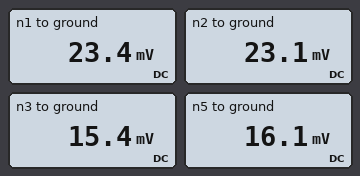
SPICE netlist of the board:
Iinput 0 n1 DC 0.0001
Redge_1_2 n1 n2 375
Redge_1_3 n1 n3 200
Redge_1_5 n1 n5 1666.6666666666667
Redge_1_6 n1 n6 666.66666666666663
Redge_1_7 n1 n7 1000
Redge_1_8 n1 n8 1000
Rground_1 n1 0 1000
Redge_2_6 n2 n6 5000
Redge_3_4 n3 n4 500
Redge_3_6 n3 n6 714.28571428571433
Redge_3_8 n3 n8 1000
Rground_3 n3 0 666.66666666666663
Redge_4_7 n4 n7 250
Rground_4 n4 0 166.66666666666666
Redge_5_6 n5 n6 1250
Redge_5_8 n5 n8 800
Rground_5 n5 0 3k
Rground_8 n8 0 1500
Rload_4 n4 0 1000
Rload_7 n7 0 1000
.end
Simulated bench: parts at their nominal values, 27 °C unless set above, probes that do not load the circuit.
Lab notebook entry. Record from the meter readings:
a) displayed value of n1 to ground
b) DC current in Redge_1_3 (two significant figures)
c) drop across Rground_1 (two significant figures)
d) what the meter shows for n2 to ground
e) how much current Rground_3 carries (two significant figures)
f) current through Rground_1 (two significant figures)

23.4 mV
40 µA
23 mV
23.1 mV
23 µA
23 µA
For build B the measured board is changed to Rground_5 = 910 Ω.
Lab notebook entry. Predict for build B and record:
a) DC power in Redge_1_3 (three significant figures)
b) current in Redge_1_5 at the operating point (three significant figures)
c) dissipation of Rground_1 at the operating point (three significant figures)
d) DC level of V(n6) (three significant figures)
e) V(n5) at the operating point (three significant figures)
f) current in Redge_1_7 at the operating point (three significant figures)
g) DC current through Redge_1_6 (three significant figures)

301 nW
6.31 µA
482 nW
17.0 mV
11.4 mV
15.5 µA
7.44 µA
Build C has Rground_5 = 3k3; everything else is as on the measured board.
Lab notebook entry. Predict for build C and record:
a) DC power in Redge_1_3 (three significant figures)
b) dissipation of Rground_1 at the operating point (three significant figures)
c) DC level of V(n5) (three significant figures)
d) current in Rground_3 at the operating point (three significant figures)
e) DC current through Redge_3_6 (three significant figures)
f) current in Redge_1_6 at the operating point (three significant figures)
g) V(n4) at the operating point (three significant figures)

322 nW
550 nW
16.3 mV
23.1 µA
5.14 µA
6.53 µA
4.50 mV
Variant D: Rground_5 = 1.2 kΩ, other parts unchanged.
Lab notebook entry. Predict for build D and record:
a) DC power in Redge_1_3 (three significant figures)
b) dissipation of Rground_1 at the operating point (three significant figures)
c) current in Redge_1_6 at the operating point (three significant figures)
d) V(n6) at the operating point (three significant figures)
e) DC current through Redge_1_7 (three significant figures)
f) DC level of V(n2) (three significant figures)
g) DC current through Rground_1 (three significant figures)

306 nW
499 nW
7.20 µA
17.5 mV
15.8 µA
22.0 mV
22.3 µA
